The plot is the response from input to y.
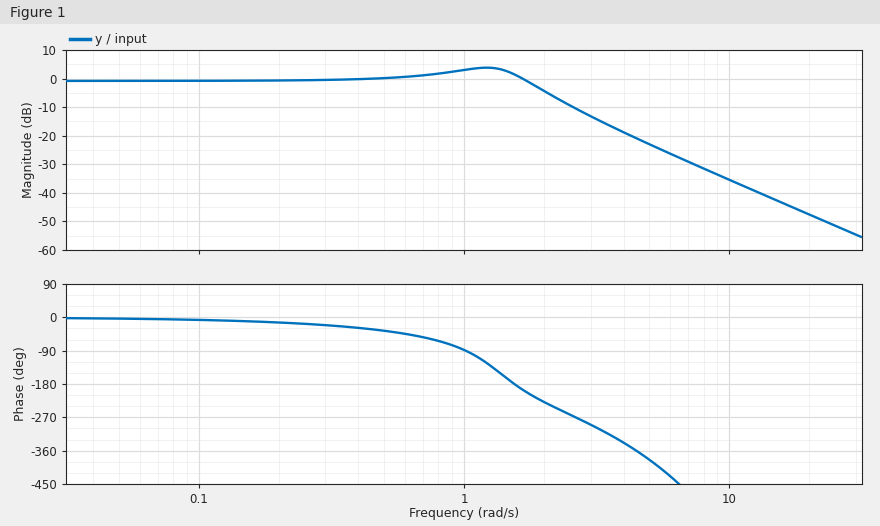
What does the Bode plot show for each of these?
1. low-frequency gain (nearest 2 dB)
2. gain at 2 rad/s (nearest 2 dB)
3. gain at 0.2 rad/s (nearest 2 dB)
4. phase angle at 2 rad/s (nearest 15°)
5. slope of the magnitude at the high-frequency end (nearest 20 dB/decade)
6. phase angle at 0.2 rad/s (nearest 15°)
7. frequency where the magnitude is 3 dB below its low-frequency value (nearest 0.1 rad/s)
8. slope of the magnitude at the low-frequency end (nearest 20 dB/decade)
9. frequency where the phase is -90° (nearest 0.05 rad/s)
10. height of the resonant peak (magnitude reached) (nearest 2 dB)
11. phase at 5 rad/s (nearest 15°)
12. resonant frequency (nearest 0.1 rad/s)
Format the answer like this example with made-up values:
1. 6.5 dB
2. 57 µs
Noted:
1. 0 dB
2. -4 dB
3. 0 dB
4. -225°
5. -40 dB/decade
6. -15°
7. 2.0 rad/s
8. 0 dB/decade
9. 1.00 rad/s
10. 4 dB
11. -390°
12. 1.2 rad/s
